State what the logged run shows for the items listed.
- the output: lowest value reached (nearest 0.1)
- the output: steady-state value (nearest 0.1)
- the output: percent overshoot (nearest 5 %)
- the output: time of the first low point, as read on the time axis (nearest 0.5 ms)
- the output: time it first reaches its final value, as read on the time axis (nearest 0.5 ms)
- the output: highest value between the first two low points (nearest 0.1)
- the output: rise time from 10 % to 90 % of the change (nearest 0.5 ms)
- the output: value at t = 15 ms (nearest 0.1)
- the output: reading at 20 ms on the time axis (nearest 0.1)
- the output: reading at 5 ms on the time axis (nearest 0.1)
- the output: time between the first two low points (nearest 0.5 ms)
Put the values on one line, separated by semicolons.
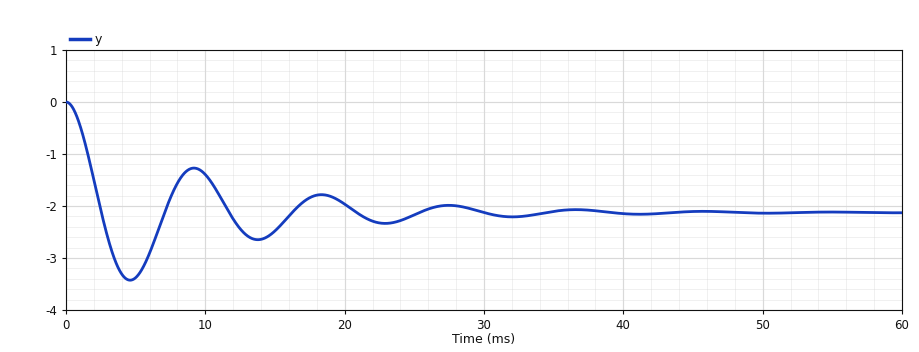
-3.4; -2.1; 60 %; 4.5 ms; 2.5 ms; -1.3; 1.5 ms; -2.5; -2.0; -3.4; 9.0 ms
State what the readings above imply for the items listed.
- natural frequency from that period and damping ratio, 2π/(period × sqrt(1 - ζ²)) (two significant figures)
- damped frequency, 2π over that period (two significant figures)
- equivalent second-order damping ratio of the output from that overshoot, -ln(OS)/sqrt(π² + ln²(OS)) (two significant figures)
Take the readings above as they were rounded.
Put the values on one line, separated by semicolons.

0.71 rad/ms; 0.70 rad/ms; 0.16
